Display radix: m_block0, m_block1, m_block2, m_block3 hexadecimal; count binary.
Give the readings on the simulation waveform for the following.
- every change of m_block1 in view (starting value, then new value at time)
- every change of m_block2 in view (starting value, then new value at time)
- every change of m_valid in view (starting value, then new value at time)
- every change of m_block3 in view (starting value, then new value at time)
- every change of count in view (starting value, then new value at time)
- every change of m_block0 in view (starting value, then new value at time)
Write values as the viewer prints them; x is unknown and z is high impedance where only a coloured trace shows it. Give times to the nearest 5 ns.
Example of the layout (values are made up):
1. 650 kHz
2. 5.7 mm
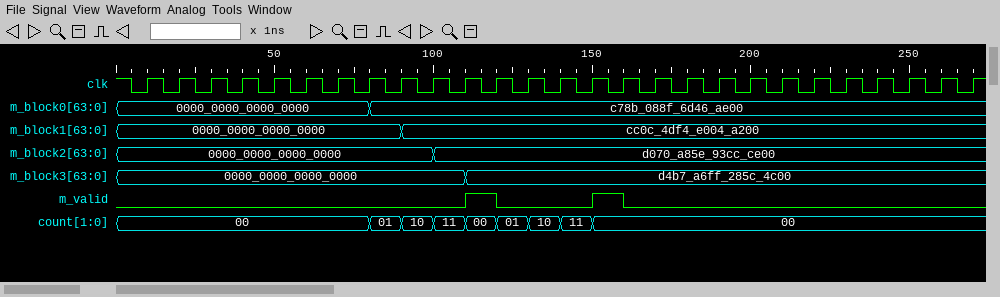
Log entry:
1. 0000_0000_0000_0000, cc0c_4df4_e004_a200 at 90 ns
2. 0000_0000_0000_0000, d070_a85e_93cc_ce00 at 100 ns
3. 0, 1 at 110 ns, 0 at 120 ns, 1 at 150 ns, 0 at 160 ns
4. 0000_0000_0000_0000, d4b7_a6ff_285c_4c00 at 110 ns
5. 00, 01 at 80 ns, 10 at 90 ns, 11 at 100 ns, 00 at 110 ns, 01 at 120 ns, 10 at 130 ns, 11 at 140 ns, 00 at 150 ns
6. 0000_0000_0000_0000, c78b_088f_6d46_ae00 at 80 ns
